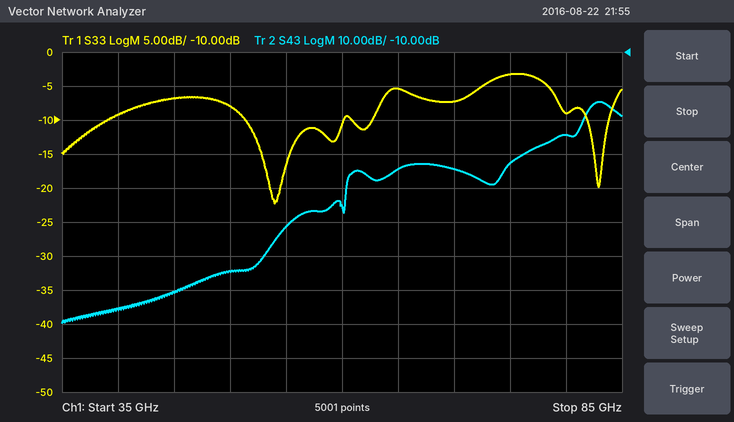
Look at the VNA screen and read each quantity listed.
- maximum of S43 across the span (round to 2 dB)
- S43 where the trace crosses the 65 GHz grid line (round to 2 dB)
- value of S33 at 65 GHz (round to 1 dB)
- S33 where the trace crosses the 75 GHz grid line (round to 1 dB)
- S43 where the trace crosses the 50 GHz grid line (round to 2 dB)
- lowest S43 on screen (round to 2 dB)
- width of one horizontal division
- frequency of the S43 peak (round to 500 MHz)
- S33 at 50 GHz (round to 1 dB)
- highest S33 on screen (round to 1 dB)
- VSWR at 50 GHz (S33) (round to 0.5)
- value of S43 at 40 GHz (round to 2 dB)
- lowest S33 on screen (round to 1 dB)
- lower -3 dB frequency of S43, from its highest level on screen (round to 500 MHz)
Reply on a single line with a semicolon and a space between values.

-24 dB; -44 dB; -5 dB; -3 dB; -74 dB; -90 dB; 5 GHz; 83.0 GHz; -8 dB; -3 dB; 2.5; -86 dB; -22 dB; 82.0 GHz
